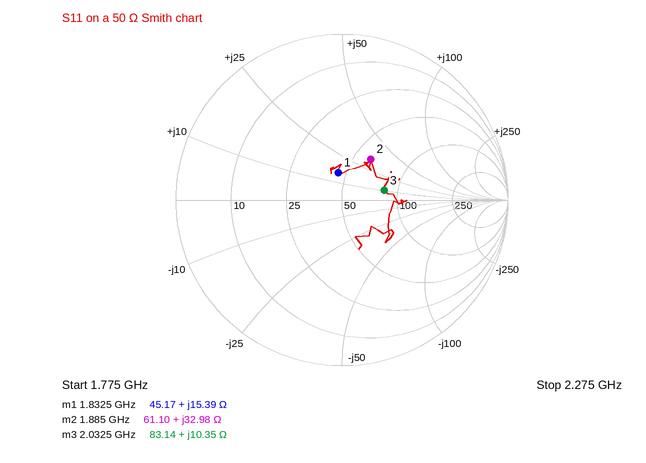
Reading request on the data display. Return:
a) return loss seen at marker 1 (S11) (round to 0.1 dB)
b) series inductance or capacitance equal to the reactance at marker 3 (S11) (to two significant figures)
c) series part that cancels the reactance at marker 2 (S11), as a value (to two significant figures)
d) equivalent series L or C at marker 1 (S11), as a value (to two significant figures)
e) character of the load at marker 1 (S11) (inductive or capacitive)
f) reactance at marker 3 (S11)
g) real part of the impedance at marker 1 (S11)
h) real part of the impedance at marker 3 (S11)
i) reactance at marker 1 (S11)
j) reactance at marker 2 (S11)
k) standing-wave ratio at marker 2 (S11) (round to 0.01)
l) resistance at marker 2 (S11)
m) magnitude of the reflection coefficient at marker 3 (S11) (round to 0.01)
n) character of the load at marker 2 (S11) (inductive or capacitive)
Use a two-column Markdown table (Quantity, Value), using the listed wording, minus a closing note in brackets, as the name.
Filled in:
| Quantity | Value |
|---|---|
| return loss seen at marker 1 (S11) | 15.5 dB |
| series inductance or capacitance equal to the reactance at marker 3 (S11) | 810 pH |
| series part that cancels the reactance at marker 2 (S11), as a value | 2.6 pF |
| equivalent series L or C at marker 1 (S11), as a value | 1.3 nH |
| character of the load at marker 1 (S11) | inductive |
| reactance at marker 3 | +10.35 Ω |
| real part of the impedance at marker 1 | 45.17 Ω |
| real part of the impedance at marker 3 | 83.14 Ω |
| reactance at marker 1 | +15.39 Ω |
| reactance at marker 2 | +32.98 Ω |
| standing-wave ratio at marker 2 (S11) | 1.86 |
| resistance at marker 2 | 61.10 Ω |
| magnitude of the reflection coefficient at marker 3 (S11) | 0.26 |
| character of the load at marker 2 (S11) | inductive |
